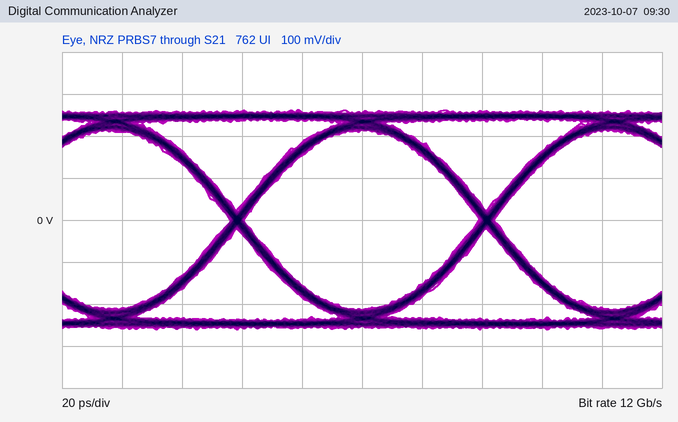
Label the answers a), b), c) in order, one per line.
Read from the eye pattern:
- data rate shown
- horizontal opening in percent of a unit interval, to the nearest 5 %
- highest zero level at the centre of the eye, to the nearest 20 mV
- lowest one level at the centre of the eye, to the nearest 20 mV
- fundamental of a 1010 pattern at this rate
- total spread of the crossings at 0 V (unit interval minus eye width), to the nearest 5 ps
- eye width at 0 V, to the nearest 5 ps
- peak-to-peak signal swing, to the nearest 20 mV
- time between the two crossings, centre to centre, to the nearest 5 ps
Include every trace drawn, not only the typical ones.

a) 12 Gb/s
b) 95 %
c) -220 mV
d) 220 mV
e) 6 GHz
f) 5 ps
g) 80 ps
h) 520 mV
i) 85 ps
